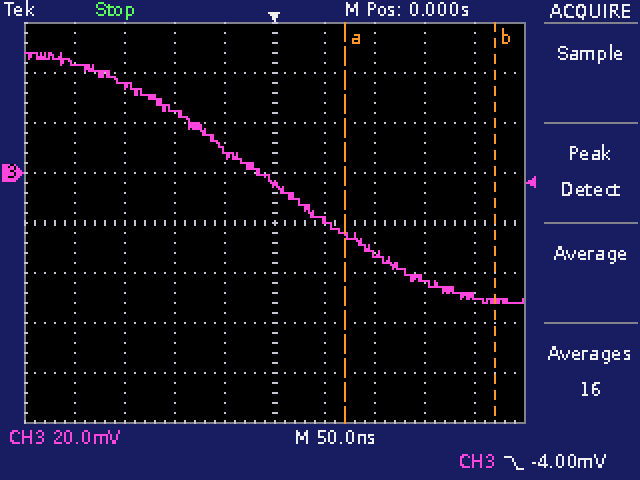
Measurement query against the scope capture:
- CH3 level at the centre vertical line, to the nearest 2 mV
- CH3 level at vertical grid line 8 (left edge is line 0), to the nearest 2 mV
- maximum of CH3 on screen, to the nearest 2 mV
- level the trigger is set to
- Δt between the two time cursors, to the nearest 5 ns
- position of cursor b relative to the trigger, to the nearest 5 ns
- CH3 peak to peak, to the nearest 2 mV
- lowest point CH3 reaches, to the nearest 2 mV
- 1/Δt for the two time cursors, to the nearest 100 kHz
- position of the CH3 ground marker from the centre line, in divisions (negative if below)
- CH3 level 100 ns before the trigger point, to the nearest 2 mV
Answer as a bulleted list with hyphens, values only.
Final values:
- -4 mV
- -42 mV
- 48 mV
- -4.00 mV
- 150 ns
- +220 ns
- 100 mV
- -52 mV
- 6.7 MHz
- +1.0 div
- 24 mV
